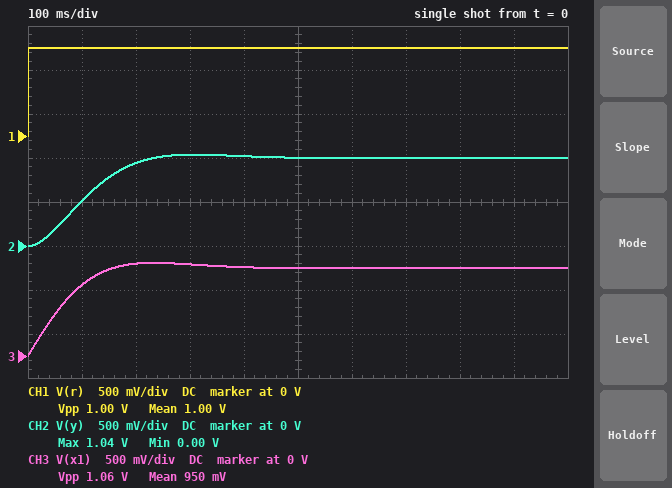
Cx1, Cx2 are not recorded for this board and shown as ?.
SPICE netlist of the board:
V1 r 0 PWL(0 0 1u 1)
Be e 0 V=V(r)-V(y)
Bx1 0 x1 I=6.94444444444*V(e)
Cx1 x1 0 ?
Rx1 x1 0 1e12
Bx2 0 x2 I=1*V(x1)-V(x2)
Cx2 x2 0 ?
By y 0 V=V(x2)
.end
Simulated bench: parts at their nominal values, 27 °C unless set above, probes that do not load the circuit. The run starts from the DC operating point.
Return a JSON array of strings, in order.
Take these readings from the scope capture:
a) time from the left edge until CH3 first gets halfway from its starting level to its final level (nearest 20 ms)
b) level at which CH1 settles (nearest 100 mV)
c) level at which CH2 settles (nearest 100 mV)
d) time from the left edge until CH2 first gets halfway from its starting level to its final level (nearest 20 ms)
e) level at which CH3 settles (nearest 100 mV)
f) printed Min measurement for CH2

["60 ms", "1.0 V", "1.0 V", "100 ms", "1.0 V", "0.00 V"]
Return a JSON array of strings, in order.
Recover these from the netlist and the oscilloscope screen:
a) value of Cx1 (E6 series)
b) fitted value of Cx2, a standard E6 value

["680 mF", "47 mF"]
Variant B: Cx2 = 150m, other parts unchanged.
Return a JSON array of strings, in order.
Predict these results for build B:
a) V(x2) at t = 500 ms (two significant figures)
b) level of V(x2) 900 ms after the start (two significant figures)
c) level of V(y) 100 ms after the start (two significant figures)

["1.2 V", "950 mV", "260 mV"]
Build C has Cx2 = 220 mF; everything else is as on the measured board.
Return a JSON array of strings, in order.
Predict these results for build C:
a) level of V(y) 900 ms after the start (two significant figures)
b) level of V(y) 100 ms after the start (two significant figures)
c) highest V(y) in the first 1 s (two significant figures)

["910 mV", "190 mV", "1.3 V"]
